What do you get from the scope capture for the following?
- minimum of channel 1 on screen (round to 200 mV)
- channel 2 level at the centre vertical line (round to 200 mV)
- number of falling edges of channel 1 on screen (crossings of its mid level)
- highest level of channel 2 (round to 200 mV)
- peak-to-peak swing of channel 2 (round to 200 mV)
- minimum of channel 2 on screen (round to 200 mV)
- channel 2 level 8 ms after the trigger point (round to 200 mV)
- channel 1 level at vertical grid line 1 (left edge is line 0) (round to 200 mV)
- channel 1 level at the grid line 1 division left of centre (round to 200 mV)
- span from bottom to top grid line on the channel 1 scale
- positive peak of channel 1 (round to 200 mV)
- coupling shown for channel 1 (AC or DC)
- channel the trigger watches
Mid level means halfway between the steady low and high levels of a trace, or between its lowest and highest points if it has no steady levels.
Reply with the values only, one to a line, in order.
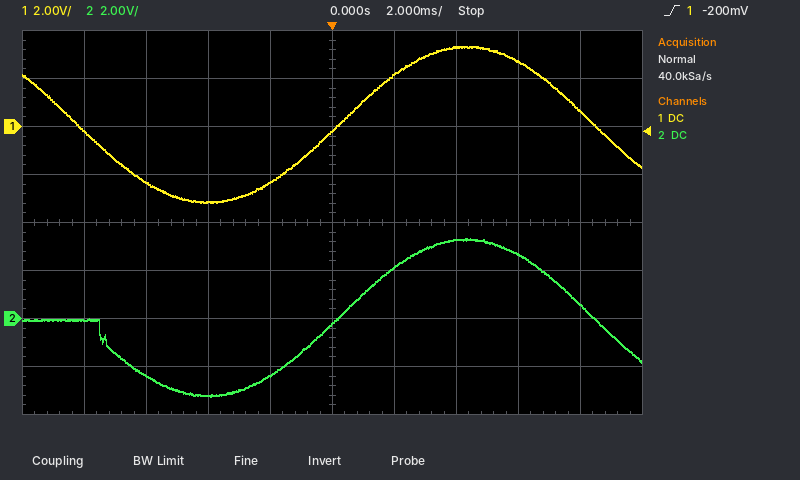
-3.2 V
-200 mV
2
3.4 V
6.6 V
-3.2 V
600 mV
-200 mV
-2.4 V
16 V
3.4 V
DC
channel 1
